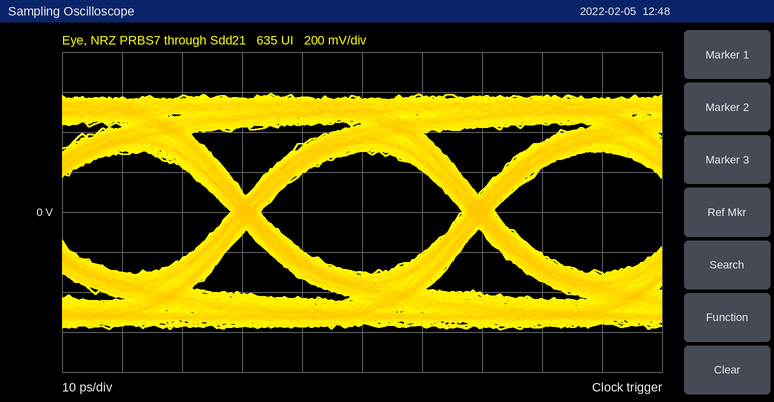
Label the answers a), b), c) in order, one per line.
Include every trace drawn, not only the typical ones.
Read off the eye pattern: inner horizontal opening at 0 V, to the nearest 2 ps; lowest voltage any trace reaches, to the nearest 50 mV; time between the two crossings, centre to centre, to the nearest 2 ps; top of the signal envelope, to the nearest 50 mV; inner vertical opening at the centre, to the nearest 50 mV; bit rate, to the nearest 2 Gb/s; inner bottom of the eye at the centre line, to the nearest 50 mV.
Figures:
a) 34 ps
b) -600 mV
c) 38 ps
d) 600 mV
e) 600 mV
f) 26 Gb/s
g) -300 mV
